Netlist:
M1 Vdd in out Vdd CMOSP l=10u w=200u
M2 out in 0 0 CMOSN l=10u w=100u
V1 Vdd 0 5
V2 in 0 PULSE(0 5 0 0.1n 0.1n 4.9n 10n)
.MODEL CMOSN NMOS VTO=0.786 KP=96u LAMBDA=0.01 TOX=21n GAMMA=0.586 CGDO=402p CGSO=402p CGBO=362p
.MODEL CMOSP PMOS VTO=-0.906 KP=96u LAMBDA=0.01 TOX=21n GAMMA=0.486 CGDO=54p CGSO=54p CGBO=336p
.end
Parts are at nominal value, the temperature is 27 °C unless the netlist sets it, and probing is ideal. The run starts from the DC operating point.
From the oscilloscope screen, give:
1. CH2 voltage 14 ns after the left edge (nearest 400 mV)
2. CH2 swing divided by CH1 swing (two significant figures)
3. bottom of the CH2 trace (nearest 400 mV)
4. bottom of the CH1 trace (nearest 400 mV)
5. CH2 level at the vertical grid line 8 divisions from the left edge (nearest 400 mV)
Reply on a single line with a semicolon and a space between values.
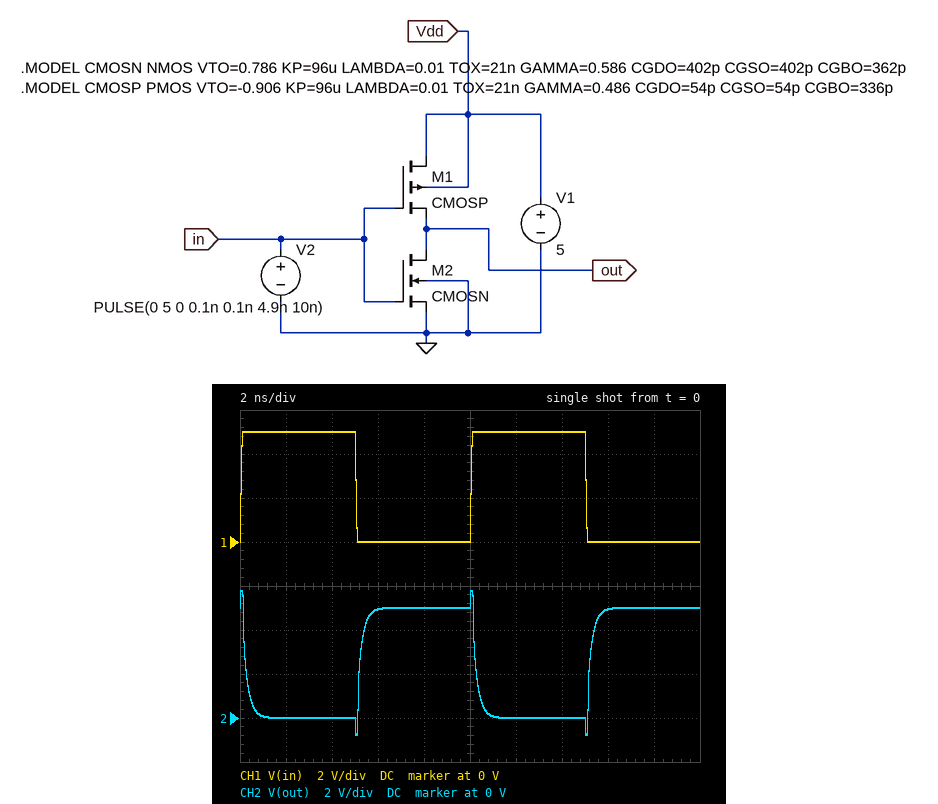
0 V; 1.3; -800 mV; 0 V; 4.8 V
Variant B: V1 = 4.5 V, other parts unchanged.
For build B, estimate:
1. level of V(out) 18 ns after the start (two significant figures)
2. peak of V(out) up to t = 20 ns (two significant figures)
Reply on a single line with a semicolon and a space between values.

4.5 V; 5.3 V
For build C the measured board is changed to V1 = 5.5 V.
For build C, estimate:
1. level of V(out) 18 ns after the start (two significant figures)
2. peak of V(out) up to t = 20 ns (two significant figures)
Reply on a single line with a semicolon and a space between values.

5.5 V; 6.3 V
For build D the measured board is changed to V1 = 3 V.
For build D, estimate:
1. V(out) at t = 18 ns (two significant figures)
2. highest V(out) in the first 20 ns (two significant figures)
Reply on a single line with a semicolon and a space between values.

3.0 V; 3.8 V
